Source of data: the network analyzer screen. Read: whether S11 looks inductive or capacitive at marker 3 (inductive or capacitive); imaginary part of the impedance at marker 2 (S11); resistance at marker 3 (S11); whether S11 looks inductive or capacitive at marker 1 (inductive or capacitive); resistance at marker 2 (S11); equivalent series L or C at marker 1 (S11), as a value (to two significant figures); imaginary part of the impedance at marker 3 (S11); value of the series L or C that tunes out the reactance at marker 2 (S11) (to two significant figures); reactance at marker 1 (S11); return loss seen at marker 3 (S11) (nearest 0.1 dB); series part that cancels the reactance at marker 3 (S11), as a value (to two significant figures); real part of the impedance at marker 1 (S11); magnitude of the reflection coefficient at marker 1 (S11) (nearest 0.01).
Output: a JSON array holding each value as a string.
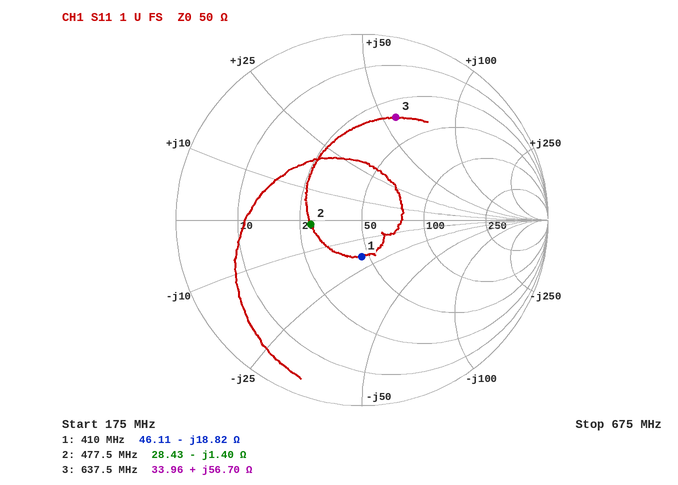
["inductive", "-1.40 Ω", "33.96 Ω", "capacitive", "28.43 Ω", "21 pF", "+56.70 Ω", "470 pH", "-18.82 Ω", "4.7 dB", "4.4 pF", "46.11 Ω", "0.20"]
